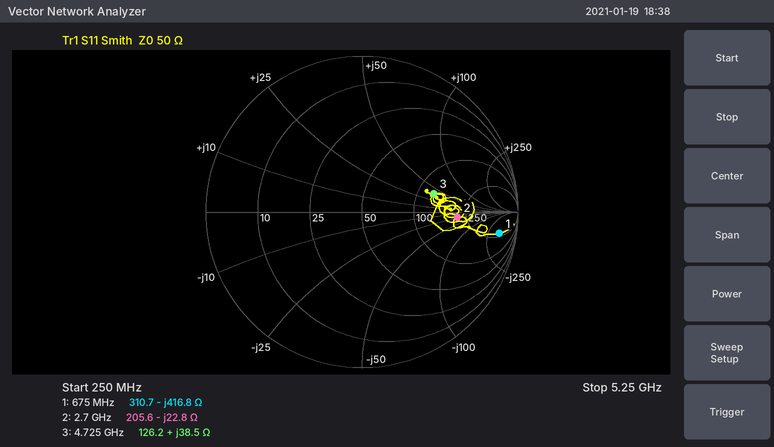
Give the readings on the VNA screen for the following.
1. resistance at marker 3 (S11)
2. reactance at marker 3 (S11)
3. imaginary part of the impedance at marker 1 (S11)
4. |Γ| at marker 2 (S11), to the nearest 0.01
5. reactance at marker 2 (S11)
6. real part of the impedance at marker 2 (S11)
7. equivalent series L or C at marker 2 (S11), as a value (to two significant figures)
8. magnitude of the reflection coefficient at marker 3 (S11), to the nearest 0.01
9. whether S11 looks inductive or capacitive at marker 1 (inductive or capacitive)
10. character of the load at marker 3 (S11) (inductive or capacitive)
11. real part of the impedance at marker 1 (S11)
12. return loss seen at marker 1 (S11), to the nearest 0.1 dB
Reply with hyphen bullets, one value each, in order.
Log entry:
- 126.2 Ω
- +38.5 Ω
- -416.8 Ω
- 0.61
- -22.8 Ω
- 205.6 Ω
- 2.6 pF
- 0.47
- capacitive
- inductive
- 310.7 Ω
- 1.0 dB
